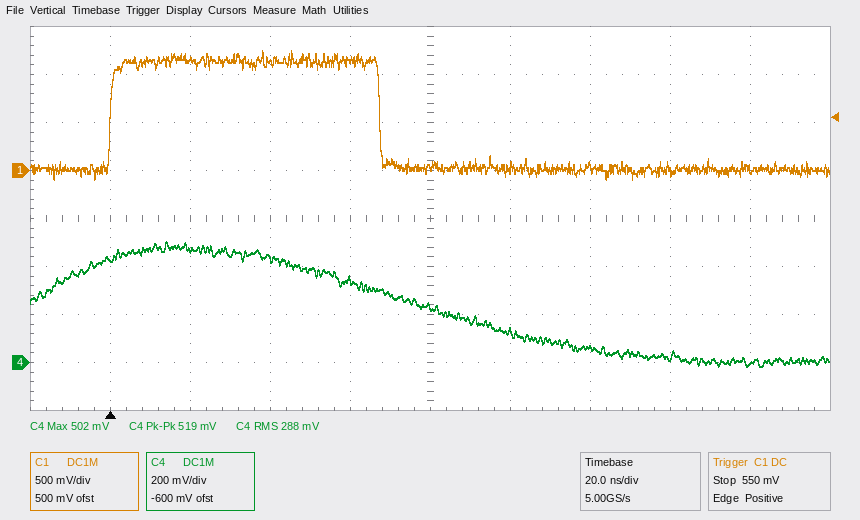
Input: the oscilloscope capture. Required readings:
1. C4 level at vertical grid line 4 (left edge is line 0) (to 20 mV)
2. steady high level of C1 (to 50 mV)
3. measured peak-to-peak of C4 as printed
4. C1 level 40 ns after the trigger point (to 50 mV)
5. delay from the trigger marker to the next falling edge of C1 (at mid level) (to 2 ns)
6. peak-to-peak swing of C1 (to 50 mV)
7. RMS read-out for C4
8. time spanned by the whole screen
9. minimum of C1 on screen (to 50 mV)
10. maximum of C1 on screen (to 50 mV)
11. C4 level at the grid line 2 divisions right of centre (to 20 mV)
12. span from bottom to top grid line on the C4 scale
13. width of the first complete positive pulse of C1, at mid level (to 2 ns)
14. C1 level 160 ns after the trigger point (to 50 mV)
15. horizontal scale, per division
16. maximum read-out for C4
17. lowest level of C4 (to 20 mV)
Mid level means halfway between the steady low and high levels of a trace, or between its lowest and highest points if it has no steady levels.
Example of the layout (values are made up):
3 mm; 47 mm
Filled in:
340 mV; 1.15 V; 519 mV; 1.15 V; 68 ns; 1.35 V; 288 mV; 200 ns; -100 mV; 1.25 V; 60 mV; 1.6 V; 68 ns; 0 mV; 20 ns; 502 mV; -20 mV
